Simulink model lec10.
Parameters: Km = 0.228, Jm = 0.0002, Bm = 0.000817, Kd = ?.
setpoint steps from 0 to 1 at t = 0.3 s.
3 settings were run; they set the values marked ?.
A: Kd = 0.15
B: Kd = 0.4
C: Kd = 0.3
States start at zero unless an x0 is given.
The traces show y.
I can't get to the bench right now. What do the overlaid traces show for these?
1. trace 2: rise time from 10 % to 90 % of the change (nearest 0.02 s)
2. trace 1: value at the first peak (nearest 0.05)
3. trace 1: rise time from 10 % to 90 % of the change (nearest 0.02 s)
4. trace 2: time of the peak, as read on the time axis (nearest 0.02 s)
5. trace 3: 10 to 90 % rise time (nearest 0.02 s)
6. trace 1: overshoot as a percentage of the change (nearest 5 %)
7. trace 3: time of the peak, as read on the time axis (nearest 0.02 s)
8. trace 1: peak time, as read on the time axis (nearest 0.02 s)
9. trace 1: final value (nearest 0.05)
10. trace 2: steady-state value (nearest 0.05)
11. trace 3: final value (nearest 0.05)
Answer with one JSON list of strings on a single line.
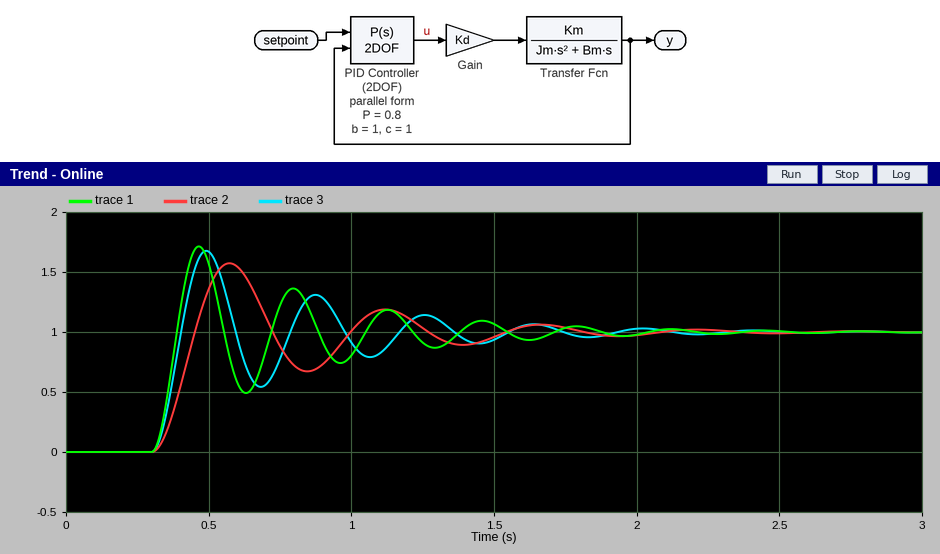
["0.10 s", "1.70", "0.06 s", "0.58 s", "0.06 s", "70 %", "0.50 s", "0.46 s", "1.00", "1.00", "1.00"]
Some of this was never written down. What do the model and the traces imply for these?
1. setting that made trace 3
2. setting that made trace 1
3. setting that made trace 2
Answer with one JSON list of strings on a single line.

["C", "B", "A"]
